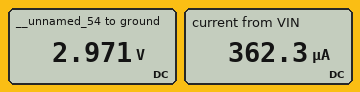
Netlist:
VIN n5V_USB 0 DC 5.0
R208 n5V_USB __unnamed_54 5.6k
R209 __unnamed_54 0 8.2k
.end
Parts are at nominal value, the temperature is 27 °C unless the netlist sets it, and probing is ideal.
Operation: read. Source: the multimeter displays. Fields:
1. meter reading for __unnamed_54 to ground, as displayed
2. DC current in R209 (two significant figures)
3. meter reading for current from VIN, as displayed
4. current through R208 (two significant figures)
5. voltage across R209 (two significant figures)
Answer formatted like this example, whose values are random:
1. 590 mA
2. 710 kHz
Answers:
1. 2.971 V
2. 360 µA
3. 362.3 µA
4. 360 µA
5. 3.0 V
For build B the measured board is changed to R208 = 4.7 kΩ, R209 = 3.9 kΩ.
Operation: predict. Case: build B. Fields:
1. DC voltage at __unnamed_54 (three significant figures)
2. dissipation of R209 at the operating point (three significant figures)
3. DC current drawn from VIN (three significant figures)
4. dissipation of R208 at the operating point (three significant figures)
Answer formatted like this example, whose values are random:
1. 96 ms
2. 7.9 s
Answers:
1. 2.27 V
2. 1.32 mW
3. 581 µA
4. 1.59 mW
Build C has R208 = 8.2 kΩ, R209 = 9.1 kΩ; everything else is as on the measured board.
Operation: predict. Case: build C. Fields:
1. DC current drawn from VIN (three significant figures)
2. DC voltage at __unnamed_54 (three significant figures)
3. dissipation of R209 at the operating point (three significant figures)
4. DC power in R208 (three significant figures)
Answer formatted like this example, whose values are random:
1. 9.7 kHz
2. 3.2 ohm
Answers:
1. 289 µA
2. 2.63 V
3. 760 µW
4. 685 µW
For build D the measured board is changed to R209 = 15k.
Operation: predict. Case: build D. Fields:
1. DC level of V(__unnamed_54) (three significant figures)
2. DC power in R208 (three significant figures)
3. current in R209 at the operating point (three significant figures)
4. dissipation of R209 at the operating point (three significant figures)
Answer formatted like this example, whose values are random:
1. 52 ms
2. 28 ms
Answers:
1. 3.64 V
2. 330 µW
3. 243 µA
4. 884 µW
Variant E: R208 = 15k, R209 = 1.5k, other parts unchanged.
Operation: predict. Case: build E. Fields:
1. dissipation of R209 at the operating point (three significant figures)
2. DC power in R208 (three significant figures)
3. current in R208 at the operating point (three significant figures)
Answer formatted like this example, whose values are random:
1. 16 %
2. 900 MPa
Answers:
1. 138 µW
2. 1.38 mW
3. 303 µA
